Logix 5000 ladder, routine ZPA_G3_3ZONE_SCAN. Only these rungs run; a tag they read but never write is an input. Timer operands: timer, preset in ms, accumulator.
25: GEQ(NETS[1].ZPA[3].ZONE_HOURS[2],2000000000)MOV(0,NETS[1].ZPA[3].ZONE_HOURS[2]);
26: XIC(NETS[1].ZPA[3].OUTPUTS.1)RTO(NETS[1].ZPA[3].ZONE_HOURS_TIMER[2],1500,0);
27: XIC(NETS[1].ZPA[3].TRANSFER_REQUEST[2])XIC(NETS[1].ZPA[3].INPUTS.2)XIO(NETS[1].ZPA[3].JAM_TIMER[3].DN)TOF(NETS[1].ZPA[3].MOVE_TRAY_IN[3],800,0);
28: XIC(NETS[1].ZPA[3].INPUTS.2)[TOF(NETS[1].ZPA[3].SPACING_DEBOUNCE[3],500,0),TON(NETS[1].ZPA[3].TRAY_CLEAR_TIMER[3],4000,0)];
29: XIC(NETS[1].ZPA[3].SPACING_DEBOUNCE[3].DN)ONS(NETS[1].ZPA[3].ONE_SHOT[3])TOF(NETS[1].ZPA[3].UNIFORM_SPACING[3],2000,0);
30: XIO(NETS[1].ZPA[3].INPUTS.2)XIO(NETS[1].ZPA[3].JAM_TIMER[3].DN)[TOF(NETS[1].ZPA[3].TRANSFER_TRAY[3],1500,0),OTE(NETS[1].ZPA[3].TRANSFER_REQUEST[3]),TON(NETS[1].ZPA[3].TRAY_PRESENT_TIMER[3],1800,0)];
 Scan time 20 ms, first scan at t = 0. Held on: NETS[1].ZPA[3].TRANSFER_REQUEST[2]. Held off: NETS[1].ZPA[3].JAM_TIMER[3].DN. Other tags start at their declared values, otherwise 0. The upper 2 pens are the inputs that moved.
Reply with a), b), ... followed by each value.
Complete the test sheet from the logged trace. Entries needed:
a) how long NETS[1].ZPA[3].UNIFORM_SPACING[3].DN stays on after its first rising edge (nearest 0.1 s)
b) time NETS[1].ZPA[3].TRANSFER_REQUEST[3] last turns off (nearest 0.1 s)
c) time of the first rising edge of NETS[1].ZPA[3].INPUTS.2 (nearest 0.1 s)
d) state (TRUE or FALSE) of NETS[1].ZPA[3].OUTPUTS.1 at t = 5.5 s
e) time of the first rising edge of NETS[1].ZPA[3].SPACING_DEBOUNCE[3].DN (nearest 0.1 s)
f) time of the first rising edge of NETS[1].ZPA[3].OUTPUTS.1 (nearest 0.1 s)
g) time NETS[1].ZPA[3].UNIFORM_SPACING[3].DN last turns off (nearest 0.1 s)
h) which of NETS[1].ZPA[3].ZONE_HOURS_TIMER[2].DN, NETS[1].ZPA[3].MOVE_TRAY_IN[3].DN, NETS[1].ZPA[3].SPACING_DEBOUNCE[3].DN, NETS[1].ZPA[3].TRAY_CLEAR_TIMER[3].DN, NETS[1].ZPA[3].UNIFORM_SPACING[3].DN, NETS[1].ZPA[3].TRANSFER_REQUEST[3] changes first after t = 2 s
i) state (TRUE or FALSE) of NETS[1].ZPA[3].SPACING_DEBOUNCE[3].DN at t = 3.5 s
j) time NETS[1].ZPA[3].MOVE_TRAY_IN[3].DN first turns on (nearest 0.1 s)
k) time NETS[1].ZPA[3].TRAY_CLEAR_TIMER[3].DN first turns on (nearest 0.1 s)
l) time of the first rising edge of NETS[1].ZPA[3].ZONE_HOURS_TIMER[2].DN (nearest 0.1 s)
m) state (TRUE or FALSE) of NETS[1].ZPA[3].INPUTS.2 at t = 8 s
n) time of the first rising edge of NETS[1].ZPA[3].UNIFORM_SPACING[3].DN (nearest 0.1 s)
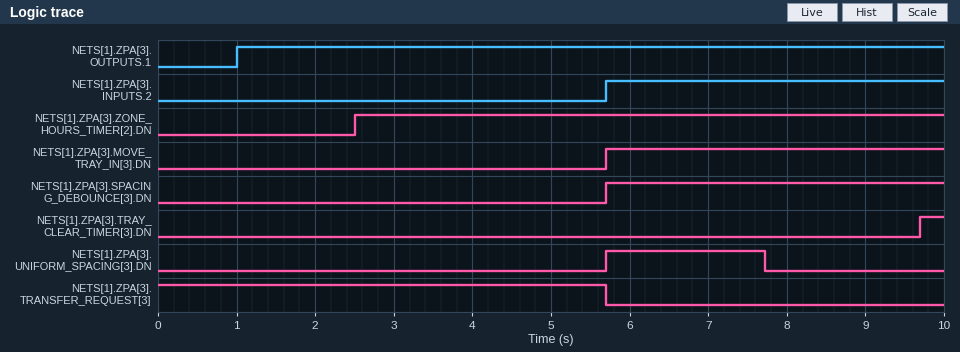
a) 2.0 s
b) 5.7 s
c) 5.7 s
d) TRUE
e) 5.7 s
f) 1.0 s
g) 7.7 s
h) NETS[1].ZPA[3].ZONE_HOURS_TIMER[2].DN
i) FALSE
j) 5.7 s
k) 9.7 s
l) 2.5 s
m) TRUE
n) 5.7 s
